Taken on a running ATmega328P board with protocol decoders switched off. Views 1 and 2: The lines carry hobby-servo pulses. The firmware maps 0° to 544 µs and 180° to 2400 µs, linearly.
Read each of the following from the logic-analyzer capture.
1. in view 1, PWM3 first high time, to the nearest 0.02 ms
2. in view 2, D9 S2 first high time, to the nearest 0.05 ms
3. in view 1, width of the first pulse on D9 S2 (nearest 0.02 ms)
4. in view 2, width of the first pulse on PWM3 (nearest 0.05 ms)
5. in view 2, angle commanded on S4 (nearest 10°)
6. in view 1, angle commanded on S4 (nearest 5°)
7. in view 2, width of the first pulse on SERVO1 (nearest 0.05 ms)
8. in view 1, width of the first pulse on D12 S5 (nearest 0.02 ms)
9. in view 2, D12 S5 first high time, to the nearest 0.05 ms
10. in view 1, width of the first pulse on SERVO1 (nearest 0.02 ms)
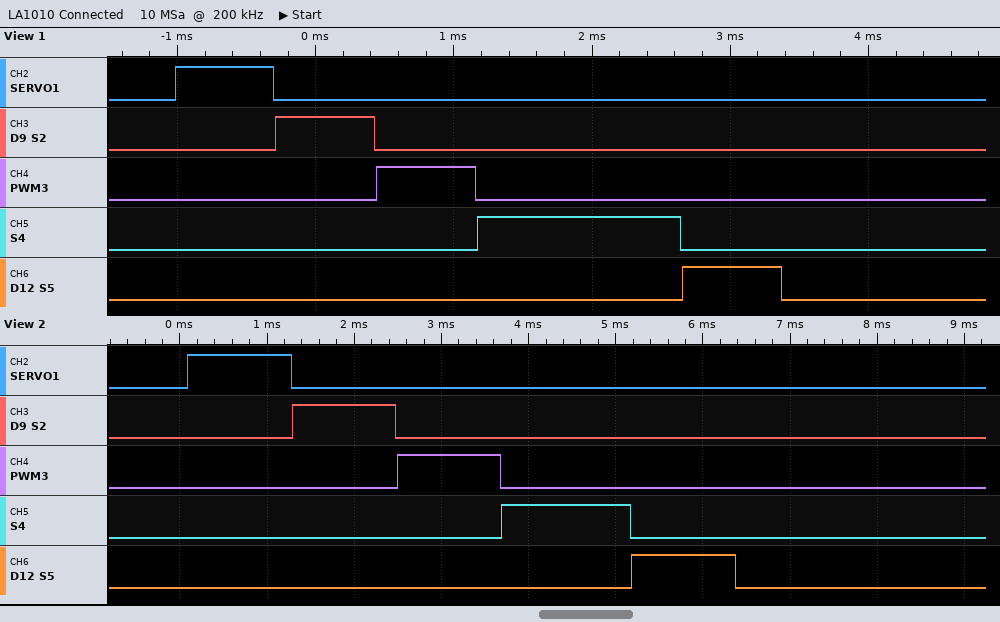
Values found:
0.72 ms
1.20 ms
0.72 ms
1.20 ms
90°
90°
1.20 ms
0.72 ms
1.20 ms
0.72 ms
